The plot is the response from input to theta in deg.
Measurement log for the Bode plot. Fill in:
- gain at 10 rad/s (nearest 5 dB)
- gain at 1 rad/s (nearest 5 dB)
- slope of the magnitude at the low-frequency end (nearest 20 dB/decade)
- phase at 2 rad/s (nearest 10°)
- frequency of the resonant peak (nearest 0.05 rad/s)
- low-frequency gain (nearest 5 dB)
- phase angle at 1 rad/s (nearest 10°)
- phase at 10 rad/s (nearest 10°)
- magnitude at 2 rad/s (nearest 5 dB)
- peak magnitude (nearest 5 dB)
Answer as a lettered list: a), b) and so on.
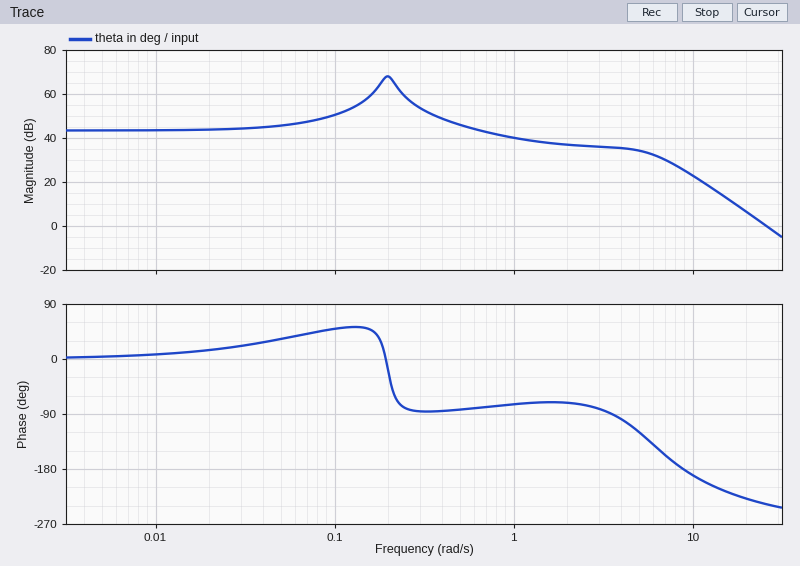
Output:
a) 25 dB
b) 40 dB
c) 0 dB/decade
d) -70°
e) 0.20 rad/s
f) 45 dB
g) -70°
h) -190°
i) 35 dB
j) 70 dB
